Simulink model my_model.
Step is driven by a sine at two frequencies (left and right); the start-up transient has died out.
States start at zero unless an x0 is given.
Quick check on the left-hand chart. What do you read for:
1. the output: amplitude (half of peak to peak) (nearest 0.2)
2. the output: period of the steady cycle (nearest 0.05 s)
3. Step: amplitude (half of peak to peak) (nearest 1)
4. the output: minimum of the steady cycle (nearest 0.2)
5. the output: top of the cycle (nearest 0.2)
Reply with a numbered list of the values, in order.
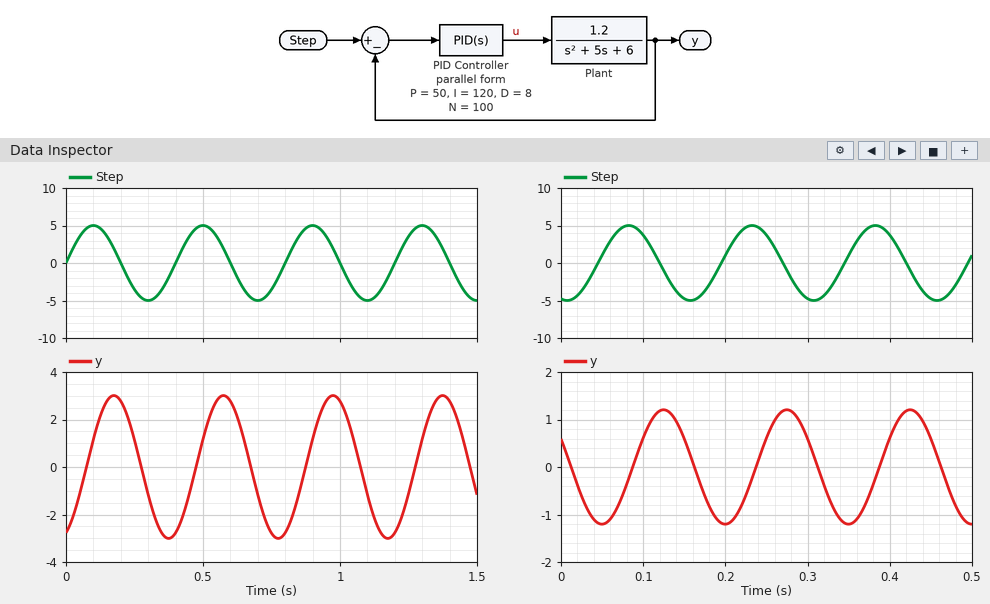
1. 3.0
2. 0.40 s
3. 5
4. -3.0
5. 3.0
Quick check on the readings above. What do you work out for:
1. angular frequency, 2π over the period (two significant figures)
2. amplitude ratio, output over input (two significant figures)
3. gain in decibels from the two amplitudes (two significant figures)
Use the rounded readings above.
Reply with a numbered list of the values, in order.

1. 16 rad/s
2. 0.60
3. -4.4 dB
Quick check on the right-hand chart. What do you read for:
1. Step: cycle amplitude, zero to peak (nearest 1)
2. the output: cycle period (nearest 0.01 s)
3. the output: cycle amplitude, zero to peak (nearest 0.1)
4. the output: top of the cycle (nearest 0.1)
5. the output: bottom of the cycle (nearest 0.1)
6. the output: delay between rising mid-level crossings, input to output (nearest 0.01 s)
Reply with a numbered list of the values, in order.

1. 5
2. 0.15 s
3. 1.2
4. 1.2
5. -1.2
6. 0.04 s
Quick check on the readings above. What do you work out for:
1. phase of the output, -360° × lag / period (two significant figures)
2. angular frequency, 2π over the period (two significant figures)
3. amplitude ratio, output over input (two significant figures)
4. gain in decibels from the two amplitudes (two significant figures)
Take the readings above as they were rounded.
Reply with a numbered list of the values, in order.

1. -96°
2. 42 rad/s
3. 0.24
4. -12 dB
